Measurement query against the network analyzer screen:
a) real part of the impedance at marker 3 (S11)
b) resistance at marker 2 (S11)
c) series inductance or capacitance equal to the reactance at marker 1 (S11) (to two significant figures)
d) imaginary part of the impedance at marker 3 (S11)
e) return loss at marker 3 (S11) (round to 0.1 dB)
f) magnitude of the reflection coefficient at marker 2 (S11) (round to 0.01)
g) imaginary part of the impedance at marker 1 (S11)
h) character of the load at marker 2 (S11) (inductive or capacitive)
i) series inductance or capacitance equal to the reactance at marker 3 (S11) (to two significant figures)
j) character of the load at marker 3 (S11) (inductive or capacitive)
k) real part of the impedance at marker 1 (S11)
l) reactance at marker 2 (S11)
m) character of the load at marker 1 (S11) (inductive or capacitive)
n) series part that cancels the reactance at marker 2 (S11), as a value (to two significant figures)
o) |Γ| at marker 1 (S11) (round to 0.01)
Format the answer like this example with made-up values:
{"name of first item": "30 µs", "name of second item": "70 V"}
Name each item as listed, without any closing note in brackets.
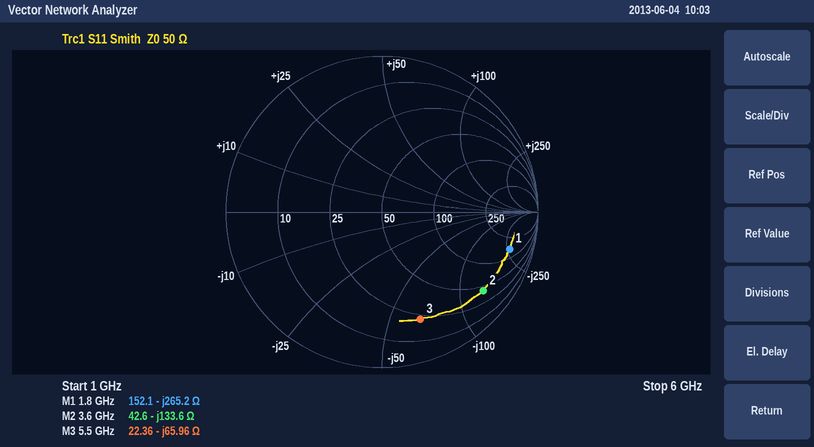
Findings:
{"real part of the impedance at marker 3": "22.36 Ω", "resistance at marker 2": "42.6 Ω", "series inductance or capacitance equal to the reactance at marker 1 (S11)": "330 fF", "imaginary part of the impedance at marker 3": "-65.96 Ω", "return loss at marker 3 (S11)": "2.7 dB", "magnitude of the reflection coefficient at marker 2 (S11)": "0.82", "imaginary part of the impedance at marker 1": "-265.2 Ω", "character of the load at marker 2 (S11)": "capacitive", "series inductance or capacitance equal to the reactance at marker 3 (S11)": "440 fF", "character of the load at marker 3 (S11)": "capacitive", "real part of the impedance at marker 1": "152.1 Ω", "reactance at marker 2": "-133.6 Ω", "character of the load at marker 1 (S11)": "capacitive", "series part that cancels the reactance at marker 2 (S11), as a value": "5.9 nH", "|Γ| at marker 1 (S11)": "0.85"}
